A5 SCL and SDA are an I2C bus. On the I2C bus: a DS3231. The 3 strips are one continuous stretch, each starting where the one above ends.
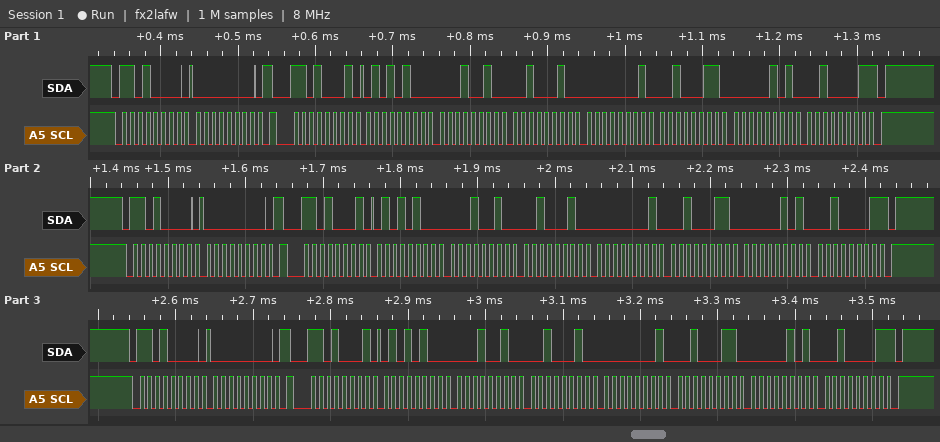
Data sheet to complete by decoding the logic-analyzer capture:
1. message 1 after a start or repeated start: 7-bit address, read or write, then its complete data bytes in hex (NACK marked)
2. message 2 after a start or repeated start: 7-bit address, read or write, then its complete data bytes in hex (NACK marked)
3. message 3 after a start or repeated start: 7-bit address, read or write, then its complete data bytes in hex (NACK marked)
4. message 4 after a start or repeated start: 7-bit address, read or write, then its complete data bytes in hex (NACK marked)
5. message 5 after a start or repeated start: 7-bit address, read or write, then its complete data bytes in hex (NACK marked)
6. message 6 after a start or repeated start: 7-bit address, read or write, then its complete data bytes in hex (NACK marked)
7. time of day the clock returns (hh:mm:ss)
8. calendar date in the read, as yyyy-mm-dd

0x68 write: 00
0x68 read: 54 12 22 01 23 05 21 NACK
0x68 write: 00
0x68 read: 54 12 22 01 23 05 21 NACK
0x68 write: 00
0x68 read: 54 12 22 01 23 05 21 NACK
22:12:54
2021-05-23
